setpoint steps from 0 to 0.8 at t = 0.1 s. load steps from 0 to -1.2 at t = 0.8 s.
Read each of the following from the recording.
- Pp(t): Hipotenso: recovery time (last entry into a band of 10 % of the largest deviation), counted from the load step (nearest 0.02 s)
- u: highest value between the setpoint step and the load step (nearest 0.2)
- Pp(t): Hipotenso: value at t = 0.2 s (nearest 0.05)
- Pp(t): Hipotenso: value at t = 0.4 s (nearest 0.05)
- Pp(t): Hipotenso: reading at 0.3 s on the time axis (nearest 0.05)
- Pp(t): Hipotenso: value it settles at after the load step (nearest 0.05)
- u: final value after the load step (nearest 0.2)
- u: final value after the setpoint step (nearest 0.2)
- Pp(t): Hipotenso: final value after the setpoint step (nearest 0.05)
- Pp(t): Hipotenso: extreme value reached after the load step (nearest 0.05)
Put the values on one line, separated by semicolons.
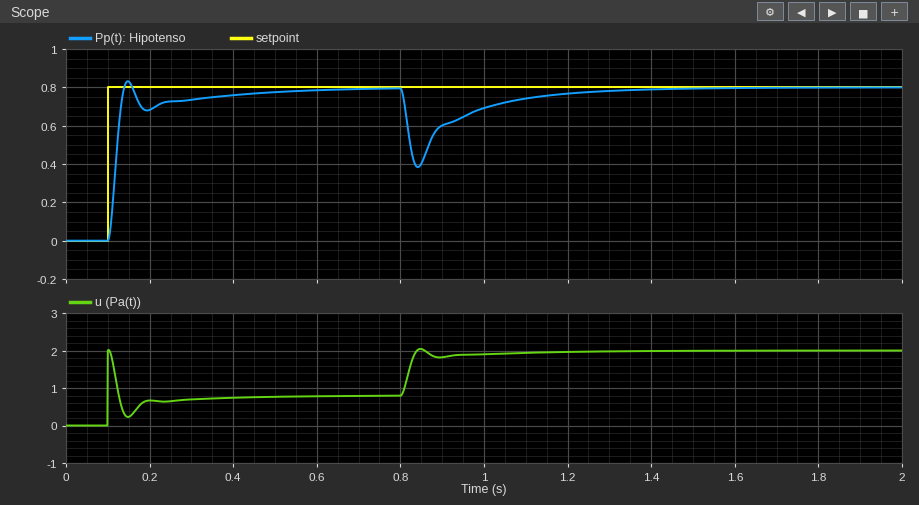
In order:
0.36 s; 2.0; 0.70; 0.75; 0.75; 0.80; 2.0; 0.8; 0.80; 0.40
